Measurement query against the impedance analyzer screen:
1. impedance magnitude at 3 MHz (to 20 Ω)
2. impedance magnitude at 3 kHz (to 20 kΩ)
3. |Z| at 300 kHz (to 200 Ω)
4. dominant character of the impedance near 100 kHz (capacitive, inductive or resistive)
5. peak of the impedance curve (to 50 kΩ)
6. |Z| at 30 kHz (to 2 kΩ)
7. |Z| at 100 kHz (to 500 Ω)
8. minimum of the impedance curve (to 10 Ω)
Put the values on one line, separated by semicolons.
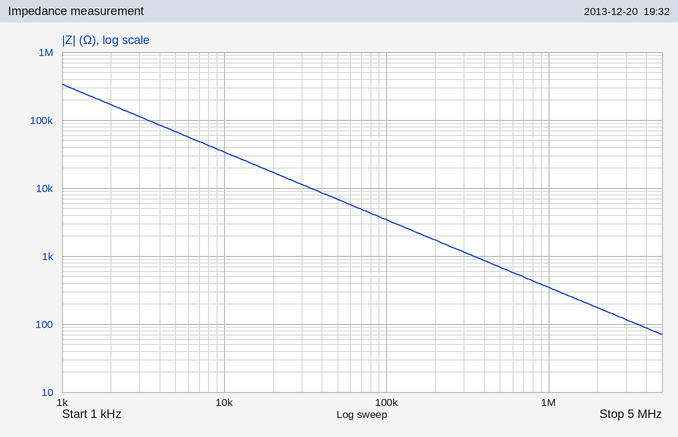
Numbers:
120 Ω; 120 kΩ; 1.2 kΩ; capacitive; 350 kΩ; 12 kΩ; 3.5 kΩ; 70 Ω
